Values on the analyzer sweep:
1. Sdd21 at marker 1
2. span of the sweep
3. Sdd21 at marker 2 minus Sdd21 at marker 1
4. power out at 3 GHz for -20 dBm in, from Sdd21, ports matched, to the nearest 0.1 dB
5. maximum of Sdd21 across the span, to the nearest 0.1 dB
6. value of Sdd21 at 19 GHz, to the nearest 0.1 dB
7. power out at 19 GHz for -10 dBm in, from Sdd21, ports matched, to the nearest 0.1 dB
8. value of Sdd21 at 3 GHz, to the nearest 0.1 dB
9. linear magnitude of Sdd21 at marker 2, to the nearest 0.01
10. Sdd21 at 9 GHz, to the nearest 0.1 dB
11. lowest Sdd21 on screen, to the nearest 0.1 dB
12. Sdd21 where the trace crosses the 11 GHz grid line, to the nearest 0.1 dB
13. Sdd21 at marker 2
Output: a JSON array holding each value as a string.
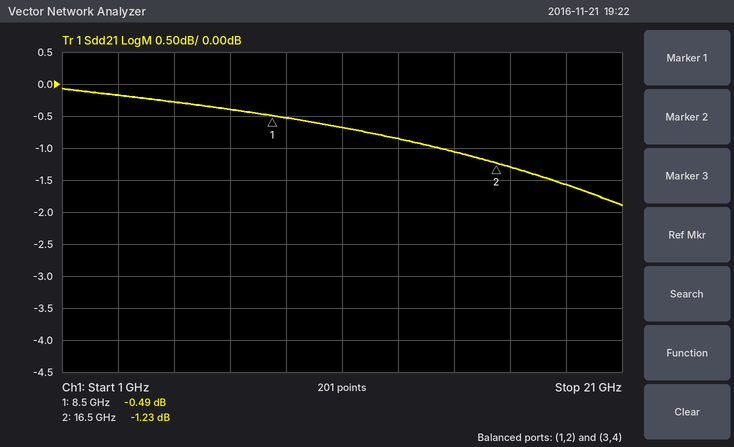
["-0.49 dB", "20 GHz", "-0.74 dB", "-20.2 dBm", "-0.1 dB", "-1.6 dB", "-11.6 dBm", "-0.2 dB", "0.87", "-0.5 dB", "-1.9 dB", "-0.7 dB", "-1.23 dB"]
